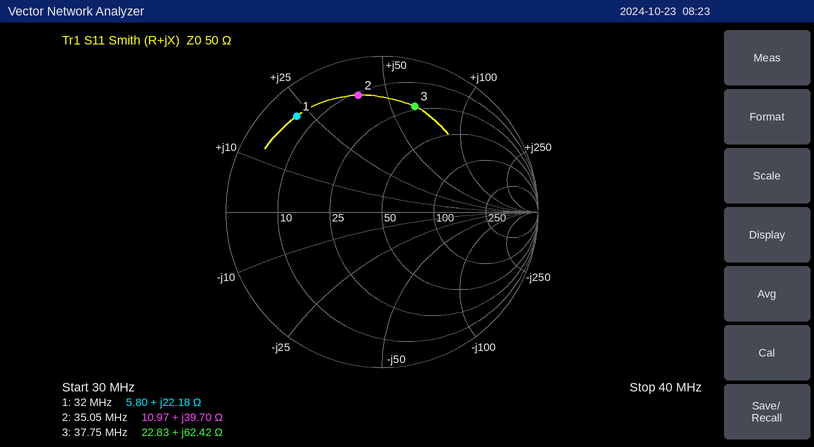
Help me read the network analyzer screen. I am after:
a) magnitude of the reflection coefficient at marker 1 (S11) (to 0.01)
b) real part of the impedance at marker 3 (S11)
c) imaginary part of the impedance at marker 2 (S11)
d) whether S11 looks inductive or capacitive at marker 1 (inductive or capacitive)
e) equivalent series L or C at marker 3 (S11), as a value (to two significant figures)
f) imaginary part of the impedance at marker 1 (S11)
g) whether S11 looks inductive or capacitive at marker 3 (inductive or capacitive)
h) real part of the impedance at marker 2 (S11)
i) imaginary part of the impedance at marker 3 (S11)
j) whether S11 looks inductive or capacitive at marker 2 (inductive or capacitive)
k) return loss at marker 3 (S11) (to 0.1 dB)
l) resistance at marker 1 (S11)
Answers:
0.82
22.83 Ω
+39.70 Ω
inductive
260 nH
+22.18 Ω
inductive
10.97 Ω
+62.42 Ω
inductive
3.0 dB
5.80 Ω
